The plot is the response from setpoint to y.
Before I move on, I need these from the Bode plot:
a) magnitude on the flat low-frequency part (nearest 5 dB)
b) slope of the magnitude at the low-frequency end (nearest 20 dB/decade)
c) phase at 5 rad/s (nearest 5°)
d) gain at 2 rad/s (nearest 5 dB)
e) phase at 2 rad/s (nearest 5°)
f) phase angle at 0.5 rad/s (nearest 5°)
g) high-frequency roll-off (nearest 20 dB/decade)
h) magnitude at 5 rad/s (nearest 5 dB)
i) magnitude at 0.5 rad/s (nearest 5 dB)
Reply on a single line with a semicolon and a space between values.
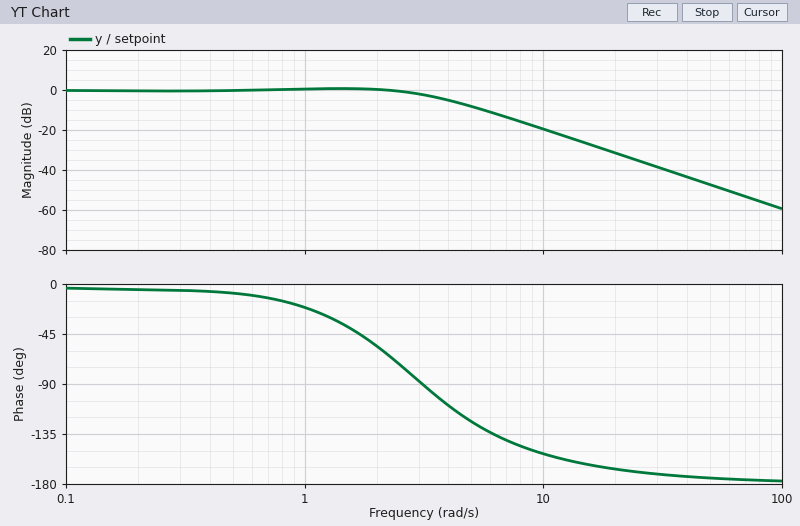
0 dB; 0 dB/decade; -125°; 0 dB; -55°; -10°; -40 dB/decade; -10 dB; 0 dB
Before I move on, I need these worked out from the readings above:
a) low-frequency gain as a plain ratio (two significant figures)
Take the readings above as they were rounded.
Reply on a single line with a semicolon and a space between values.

1.0
